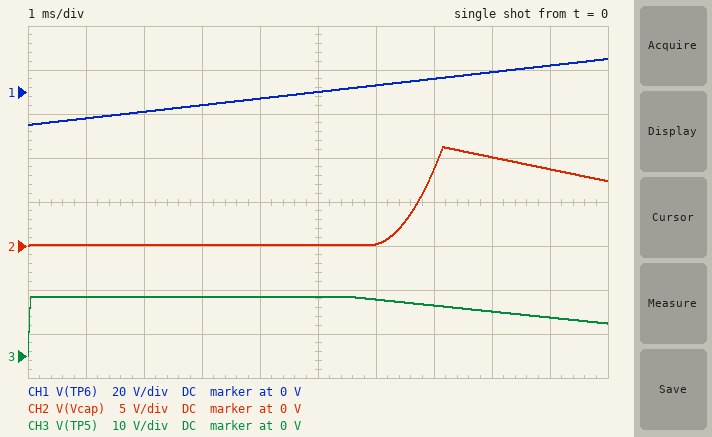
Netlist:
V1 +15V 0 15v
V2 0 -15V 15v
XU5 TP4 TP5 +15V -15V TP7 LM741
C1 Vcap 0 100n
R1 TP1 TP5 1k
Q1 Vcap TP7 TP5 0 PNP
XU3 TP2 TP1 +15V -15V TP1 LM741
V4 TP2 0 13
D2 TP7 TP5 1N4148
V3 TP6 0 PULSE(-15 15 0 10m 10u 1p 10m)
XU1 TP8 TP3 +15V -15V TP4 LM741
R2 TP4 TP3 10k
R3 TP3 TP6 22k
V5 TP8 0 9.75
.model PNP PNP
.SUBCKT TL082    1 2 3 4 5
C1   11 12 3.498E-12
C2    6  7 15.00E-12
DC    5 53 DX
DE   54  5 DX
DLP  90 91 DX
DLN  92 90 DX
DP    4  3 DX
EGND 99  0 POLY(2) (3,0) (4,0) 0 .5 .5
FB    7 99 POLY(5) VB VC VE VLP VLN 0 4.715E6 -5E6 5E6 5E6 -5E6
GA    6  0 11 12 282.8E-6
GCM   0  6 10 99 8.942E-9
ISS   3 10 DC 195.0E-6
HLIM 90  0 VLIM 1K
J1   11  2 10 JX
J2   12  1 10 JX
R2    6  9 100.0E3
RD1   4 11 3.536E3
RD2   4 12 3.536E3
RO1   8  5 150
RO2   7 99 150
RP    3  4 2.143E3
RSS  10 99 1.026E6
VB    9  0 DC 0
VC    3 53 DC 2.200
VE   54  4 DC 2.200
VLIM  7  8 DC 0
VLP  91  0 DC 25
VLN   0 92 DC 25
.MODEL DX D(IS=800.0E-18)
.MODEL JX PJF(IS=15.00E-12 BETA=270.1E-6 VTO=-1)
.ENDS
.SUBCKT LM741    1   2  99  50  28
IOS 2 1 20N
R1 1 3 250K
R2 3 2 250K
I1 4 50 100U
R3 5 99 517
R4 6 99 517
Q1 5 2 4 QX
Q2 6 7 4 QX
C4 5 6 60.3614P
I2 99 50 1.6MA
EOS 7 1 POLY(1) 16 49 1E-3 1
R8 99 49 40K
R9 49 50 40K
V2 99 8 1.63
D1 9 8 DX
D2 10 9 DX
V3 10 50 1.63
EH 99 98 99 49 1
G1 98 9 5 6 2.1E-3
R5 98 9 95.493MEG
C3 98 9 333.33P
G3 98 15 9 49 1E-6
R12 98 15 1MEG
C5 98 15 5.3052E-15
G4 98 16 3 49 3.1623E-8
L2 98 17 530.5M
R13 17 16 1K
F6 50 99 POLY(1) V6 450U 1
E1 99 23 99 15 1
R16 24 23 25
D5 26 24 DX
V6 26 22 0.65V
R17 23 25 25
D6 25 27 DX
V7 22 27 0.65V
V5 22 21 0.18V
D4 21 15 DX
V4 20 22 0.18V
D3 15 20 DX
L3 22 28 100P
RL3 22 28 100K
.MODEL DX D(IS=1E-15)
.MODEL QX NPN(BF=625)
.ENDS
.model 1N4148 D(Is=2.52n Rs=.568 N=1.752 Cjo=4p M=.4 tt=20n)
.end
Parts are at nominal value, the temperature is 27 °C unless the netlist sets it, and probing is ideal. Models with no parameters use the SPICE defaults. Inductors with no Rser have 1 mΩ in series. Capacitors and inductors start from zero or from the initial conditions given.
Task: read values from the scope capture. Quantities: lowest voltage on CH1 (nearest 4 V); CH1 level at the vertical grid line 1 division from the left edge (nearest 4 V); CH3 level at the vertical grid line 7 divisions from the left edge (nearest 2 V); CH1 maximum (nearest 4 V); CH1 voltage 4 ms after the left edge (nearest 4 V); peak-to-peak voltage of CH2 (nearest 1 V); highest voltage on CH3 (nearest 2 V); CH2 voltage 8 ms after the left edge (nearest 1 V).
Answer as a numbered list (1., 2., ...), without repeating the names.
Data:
1. -16 V
2. -12 V
3. 12 V
4. 16 V
5. -4 V
6. 11 V
7. 14 V
8. 10 V
